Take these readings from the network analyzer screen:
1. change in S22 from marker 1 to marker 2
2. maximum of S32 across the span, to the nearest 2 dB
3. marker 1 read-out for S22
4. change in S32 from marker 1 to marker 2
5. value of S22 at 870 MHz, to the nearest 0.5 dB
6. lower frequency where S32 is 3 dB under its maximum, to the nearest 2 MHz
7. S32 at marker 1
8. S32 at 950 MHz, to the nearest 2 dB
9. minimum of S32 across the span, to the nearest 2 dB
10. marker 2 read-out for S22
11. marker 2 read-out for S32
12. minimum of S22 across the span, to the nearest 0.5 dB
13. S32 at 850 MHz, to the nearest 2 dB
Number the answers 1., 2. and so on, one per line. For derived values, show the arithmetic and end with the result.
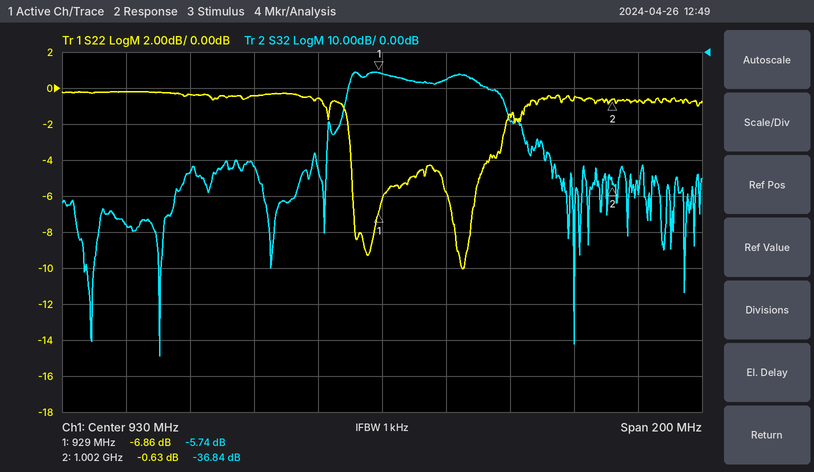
1. -0.63 − (-6.86) = 6.23 dB
2. -6 dB
3. -6.86 dB
4. -36.84 − (-5.74) = -31.10 dB
5. -0.5 dB
6. 920 MHz
7. -5.74 dB
8. -8 dB
9. -84 dB
10. -0.63 dB
11. -36.84 dB
12. -10.0 dB
13. -48 dB
